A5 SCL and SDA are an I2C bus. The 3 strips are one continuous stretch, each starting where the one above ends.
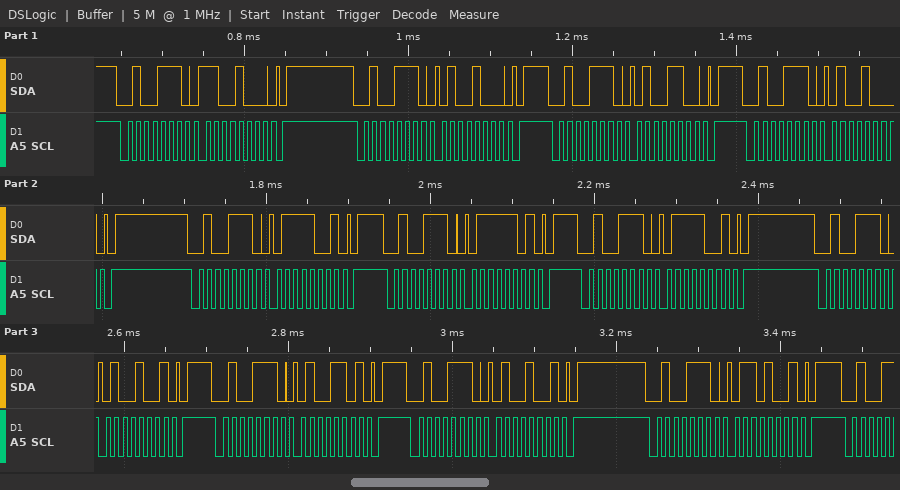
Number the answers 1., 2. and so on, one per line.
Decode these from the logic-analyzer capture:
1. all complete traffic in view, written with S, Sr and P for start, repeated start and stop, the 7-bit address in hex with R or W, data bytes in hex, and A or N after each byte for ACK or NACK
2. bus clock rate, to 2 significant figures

1. S 27W A C8 A P S 27W A 48 A P S 27W A 4C A P S 27W A 48 A P S 27W A 79 A P S 27W A 7D A P S 27W A 79 A P S 27W A 49 A P S 27W A 4D A P S 27W A 49 A P S 27W A 69 A P
2. 100 kHz
